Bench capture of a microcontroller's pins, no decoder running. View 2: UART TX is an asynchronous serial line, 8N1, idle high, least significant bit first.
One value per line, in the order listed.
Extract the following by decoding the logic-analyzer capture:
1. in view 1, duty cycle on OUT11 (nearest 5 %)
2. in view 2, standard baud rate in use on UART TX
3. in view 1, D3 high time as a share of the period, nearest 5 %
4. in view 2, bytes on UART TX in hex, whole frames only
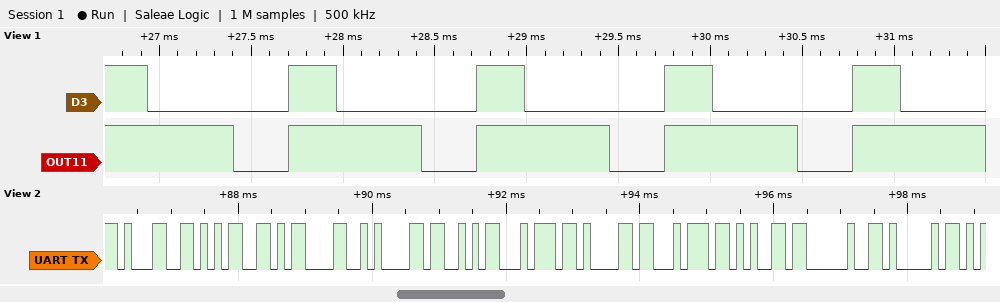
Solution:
70 %
9600 baud
25 %
0x31 0x35 0x0D 0x0A 0x53 0x74 0x61 0x74 0x65 0x20 0x41
